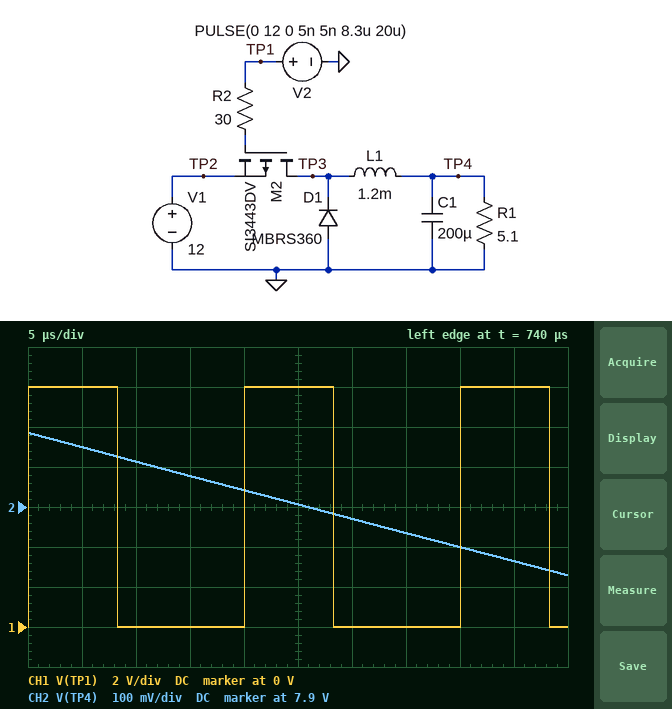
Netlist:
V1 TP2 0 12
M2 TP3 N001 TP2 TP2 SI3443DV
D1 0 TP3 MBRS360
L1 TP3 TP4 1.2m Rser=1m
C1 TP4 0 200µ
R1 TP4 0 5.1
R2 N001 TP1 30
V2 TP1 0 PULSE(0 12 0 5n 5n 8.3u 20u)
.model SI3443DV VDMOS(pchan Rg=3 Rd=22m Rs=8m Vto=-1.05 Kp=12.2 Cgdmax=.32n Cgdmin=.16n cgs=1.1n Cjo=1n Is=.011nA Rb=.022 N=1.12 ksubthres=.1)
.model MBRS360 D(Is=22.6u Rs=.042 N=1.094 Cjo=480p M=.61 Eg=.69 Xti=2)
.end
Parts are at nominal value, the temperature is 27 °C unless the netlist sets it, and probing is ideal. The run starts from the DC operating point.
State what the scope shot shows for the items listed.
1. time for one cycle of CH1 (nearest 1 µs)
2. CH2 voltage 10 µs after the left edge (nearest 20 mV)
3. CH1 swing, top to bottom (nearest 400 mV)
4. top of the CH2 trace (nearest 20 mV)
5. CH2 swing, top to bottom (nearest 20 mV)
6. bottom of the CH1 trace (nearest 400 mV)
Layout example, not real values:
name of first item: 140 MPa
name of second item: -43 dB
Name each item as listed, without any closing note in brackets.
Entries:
time for one cycle of CH1: 20 µs
CH2 voltage 10 µs after the left edge: 8.02 V
CH1 swing, top to bottom: 12.0 V
top of the CH2 trace: 8.08 V
CH2 swing, top to bottom: 360 mV
bottom of the CH1 trace: 0 V
